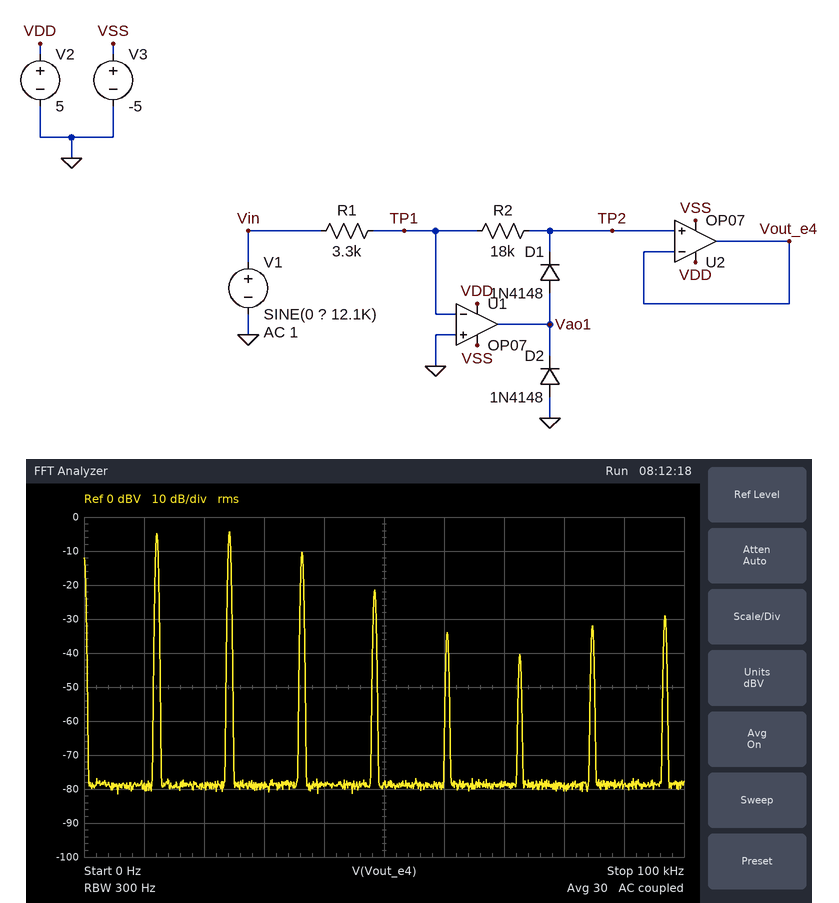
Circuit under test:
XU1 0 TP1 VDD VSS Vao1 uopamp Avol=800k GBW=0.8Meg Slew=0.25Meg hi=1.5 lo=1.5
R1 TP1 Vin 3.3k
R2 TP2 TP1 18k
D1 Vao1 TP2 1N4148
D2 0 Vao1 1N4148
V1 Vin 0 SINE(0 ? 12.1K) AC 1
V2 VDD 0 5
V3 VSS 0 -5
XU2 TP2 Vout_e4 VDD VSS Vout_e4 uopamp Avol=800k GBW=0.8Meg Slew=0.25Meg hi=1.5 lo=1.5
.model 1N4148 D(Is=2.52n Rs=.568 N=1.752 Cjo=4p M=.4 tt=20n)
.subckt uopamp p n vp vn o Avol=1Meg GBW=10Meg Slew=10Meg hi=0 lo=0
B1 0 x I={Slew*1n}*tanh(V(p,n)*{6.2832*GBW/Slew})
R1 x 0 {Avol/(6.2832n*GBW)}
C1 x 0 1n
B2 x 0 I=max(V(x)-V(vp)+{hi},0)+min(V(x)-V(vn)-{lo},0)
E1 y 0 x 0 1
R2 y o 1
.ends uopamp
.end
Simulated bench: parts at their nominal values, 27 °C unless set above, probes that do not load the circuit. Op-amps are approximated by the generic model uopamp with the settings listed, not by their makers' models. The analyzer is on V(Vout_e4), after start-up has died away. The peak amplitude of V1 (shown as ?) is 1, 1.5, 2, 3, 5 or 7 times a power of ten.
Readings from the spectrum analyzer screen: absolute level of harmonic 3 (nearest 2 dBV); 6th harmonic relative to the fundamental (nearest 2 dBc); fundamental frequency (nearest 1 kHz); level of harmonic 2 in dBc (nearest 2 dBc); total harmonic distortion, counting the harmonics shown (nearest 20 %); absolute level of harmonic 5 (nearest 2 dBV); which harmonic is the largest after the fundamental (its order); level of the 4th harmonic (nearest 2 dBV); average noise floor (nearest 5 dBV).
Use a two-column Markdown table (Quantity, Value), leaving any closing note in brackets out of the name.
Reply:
| Quantity | Value |
|---|---|
| absolute level of harmonic 3 | -10 dBV |
| 6th harmonic relative to the fundamental | -36 dBc |
| fundamental frequency | 12 kHz |
| level of harmonic 2 in dBc | 0 dBc |
| total harmonic distortion, counting the harmonics shown | 120 % |
| absolute level of harmonic 5 | -34 dBV |
| which harmonic is the largest after the fundamental | 2 |
| level of the 4th harmonic | -22 dBV |
| average noise floor | -80 dBV |
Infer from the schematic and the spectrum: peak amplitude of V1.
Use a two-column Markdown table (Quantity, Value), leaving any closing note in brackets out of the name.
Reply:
| Quantity | Value |
|---|---|
| peak amplitude of V1 | 700 mV |
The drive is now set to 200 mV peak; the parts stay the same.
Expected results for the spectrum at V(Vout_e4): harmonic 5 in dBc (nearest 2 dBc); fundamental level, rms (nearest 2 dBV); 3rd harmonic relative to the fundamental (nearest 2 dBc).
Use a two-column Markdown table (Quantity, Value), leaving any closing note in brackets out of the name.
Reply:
| Quantity | Value |
|---|---|
| harmonic 5 in dBc | -14 dBc |
| fundamental level, rms | -14 dBV |
| 3rd harmonic relative to the fundamental | -4 dBc |
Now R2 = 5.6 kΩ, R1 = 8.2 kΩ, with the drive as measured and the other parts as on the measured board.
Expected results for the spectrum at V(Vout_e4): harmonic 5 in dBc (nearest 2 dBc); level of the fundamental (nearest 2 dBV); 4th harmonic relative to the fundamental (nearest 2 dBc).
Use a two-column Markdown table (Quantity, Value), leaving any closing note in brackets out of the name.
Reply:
| Quantity | Value |
|---|---|
| harmonic 5 in dBc | -14 dBc |
| level of the fundamental | -12 dBV |
| 4th harmonic relative to the fundamental | -14 dBc |
